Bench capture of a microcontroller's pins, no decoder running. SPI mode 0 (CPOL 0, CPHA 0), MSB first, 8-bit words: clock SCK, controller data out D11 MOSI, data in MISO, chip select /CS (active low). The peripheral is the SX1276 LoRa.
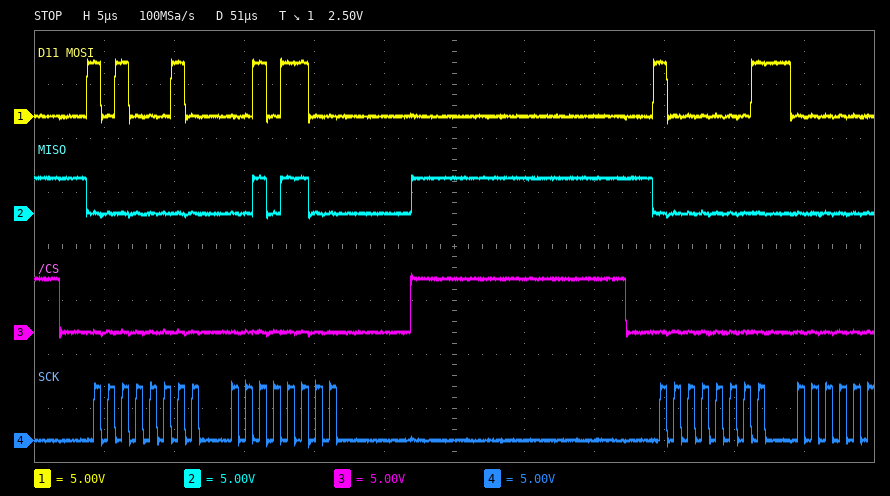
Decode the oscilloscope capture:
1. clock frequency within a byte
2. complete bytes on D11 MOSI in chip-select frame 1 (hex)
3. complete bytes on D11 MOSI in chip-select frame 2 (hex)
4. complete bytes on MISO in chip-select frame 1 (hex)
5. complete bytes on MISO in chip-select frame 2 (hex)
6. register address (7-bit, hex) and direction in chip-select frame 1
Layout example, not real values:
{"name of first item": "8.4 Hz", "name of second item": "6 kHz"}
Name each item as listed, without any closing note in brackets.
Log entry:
{"clock frequency within a byte": "1 MHz", "complete bytes on D11 MOSI in chip-select frame 1": "A2 2C", "complete bytes on D11 MOSI in chip-select frame 2": "81", "complete bytes on MISO in chip-select frame 1": "00 2C", "complete bytes on MISO in chip-select frame 2": "00", "register address (7-bit, hex) and direction in chip-select frame 1": "0x22 write"}
